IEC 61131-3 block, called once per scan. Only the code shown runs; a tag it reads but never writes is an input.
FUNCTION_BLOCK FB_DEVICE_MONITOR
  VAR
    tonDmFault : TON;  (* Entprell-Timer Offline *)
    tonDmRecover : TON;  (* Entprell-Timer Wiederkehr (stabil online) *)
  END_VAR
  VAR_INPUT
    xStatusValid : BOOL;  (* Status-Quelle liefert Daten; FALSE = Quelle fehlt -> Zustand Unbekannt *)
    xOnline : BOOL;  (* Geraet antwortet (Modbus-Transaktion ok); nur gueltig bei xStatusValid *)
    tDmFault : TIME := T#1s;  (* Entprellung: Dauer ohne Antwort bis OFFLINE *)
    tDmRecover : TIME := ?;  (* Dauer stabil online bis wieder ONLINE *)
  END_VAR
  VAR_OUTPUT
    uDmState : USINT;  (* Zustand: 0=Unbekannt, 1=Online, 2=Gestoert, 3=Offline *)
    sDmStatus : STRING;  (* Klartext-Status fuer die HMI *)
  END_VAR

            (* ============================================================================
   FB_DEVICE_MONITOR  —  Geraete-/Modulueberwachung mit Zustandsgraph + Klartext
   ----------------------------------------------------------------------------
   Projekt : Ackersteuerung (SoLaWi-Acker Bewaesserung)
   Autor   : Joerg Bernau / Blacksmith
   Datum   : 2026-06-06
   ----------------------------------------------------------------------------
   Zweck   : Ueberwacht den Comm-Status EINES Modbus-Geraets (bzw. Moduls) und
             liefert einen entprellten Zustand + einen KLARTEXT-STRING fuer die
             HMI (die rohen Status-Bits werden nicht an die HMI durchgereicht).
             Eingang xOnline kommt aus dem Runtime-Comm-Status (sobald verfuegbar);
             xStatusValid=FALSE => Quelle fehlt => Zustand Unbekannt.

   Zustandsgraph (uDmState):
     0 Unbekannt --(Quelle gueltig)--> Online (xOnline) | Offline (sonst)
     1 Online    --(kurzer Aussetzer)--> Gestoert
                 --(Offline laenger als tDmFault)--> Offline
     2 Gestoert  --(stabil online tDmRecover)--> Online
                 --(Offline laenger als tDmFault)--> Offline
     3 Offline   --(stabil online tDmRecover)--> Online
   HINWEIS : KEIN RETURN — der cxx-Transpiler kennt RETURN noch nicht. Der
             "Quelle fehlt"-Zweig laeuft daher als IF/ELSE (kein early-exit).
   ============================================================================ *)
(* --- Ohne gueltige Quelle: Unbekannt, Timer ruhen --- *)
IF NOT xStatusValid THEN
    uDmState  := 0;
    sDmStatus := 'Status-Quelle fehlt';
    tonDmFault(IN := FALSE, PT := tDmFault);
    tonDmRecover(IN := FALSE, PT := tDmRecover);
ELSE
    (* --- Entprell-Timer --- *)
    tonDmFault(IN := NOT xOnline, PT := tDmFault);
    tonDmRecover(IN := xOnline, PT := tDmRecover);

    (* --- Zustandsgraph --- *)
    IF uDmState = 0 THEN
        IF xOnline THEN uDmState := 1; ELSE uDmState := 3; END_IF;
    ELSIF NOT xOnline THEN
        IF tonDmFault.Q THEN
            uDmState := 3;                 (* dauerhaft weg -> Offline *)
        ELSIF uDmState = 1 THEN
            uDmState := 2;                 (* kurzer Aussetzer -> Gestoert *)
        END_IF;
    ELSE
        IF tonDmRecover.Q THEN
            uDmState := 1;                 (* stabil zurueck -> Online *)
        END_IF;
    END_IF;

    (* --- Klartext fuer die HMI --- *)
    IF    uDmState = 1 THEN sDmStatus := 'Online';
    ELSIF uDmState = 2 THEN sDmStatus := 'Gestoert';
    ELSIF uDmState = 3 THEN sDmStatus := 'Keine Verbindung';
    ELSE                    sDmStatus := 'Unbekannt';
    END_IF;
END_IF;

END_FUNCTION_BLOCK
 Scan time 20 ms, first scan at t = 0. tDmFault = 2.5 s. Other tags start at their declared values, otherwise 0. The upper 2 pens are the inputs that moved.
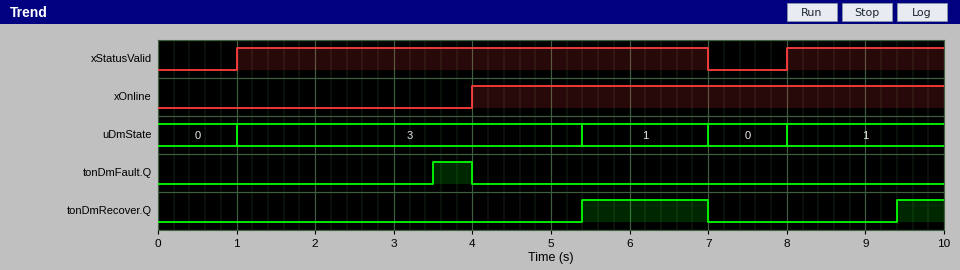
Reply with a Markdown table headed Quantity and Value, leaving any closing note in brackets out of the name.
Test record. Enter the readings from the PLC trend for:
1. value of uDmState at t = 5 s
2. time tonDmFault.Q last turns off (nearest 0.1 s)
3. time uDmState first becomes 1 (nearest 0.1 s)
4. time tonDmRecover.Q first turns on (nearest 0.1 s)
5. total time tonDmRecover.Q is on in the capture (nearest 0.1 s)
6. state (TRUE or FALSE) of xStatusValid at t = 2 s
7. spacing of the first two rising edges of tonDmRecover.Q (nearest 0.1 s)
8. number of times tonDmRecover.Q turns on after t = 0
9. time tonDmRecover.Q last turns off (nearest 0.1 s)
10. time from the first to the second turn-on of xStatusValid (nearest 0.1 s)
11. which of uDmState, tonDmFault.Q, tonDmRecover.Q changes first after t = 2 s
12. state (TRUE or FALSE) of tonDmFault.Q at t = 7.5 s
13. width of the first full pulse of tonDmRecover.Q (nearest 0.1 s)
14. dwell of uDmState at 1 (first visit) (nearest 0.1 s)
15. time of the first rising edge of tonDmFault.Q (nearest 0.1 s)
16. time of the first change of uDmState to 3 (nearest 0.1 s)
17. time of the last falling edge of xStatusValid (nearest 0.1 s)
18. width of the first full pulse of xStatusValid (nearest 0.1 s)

| Quantity | Value |
|---|---|
| value of uDmState at t = 5 s | 3 |
| time tonDmFault.Q last turns off | 4.0 s |
| time uDmState first becomes 1 | 5.4 s |
| time tonDmRecover.Q first turns on | 5.4 s |
| total time tonDmRecover.Q is on in the capture | 2.2 s |
| state (TRUE or FALSE) of xStatusValid at t = 2 s | TRUE |
| spacing of the first two rising edges of tonDmRecover.Q | 4.0 s |
| number of times tonDmRecover.Q turns on after t = 0 | 2 |
| time tonDmRecover.Q last turns off | 7.0 s |
| time from the first to the second turn-on of xStatusValid | 7.0 s |
| which of uDmState, tonDmFault.Q, tonDmRecover.Q changes first after t = 2 s | tonDmFault.Q |
| state (TRUE or FALSE) of tonDmFault.Q at t = 7.5 s | FALSE |
| width of the first full pulse of tonDmRecover.Q | 1.6 s |
| dwell of uDmState at 1 (first visit) | 1.6 s |
| time of the first rising edge of tonDmFault.Q | 3.5 s |
| time of the first change of uDmState to 3 | 1.0 s |
| time of the last falling edge of xStatusValid | 7.0 s |
| width of the first full pulse of xStatusValid | 6.0 s |
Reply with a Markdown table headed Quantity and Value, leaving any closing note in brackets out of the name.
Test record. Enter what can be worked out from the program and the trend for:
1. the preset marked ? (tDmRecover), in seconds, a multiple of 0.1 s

| Quantity | Value |
|---|---|
| the preset marked ? (tDmRecover), in seconds, a multiple of 0.1 s | 1.4 s |
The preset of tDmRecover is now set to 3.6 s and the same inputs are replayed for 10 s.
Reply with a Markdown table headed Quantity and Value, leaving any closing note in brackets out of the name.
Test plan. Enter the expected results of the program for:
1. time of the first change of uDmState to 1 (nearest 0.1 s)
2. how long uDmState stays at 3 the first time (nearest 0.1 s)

| Quantity | Value |
|---|---|
| time of the first change of uDmState to 1 | 8.0 s |
| how long uDmState stays at 3 the first time | 6.0 s |
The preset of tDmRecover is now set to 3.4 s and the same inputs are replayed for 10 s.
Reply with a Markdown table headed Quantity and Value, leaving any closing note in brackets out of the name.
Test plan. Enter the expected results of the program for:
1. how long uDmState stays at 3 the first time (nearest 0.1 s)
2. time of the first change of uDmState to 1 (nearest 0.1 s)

| Quantity | Value |
|---|---|
| how long uDmState stays at 3 the first time | 6.0 s |
| time of the first change of uDmState to 1 | 8.0 s |
